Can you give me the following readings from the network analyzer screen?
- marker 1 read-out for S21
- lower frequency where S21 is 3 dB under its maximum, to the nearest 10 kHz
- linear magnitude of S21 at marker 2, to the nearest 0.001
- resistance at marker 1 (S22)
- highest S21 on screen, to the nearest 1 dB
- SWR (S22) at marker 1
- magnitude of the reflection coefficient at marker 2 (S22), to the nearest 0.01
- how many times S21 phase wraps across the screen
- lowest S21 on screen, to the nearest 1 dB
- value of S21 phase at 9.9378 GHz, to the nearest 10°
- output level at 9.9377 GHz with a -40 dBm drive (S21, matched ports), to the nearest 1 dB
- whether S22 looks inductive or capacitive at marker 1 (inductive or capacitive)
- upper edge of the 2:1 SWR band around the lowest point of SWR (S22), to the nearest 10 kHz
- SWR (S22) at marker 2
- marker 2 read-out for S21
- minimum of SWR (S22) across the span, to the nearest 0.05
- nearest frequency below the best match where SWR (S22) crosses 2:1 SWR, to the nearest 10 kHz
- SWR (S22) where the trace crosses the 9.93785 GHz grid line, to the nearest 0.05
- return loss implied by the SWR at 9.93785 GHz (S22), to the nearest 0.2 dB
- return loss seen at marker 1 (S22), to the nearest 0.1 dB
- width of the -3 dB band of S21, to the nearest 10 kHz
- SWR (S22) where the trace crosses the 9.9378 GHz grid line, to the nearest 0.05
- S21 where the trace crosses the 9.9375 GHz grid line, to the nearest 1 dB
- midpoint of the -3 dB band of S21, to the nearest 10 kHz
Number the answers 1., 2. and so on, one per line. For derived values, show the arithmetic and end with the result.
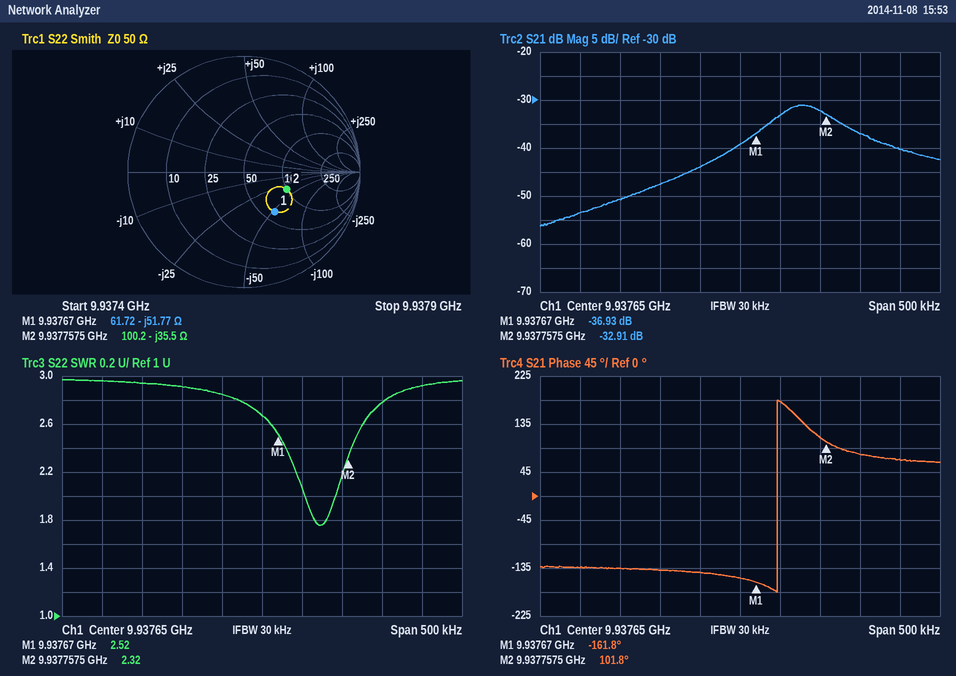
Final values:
1. -36.93 dB
2. 9.93769 GHz
3. 10^(-32.91/20) ≈ 0.023
4. 61.72 Ω
5. -31 dB
6. 2.52
7. 0.40
8. 1
9. -56 dB
10. 80°
11. -40 dBm + (-33 dB) = -73 dBm
12. capacitive
13. 9.93774 GHz
14. 2.32
15. -32.91 dB
16. 1.75
17. 9.93770 GHz
18. 2.90
19. −20 log10((2.9 − 1)/(2.9 + 1)) ≈ 6.2 dB
20. 7.3 dB
21. 9.93777 GHz − 9.93769 GHz = 80 kHz
22. 2.80
23. -51 dB
24. 9.93773 GHz
